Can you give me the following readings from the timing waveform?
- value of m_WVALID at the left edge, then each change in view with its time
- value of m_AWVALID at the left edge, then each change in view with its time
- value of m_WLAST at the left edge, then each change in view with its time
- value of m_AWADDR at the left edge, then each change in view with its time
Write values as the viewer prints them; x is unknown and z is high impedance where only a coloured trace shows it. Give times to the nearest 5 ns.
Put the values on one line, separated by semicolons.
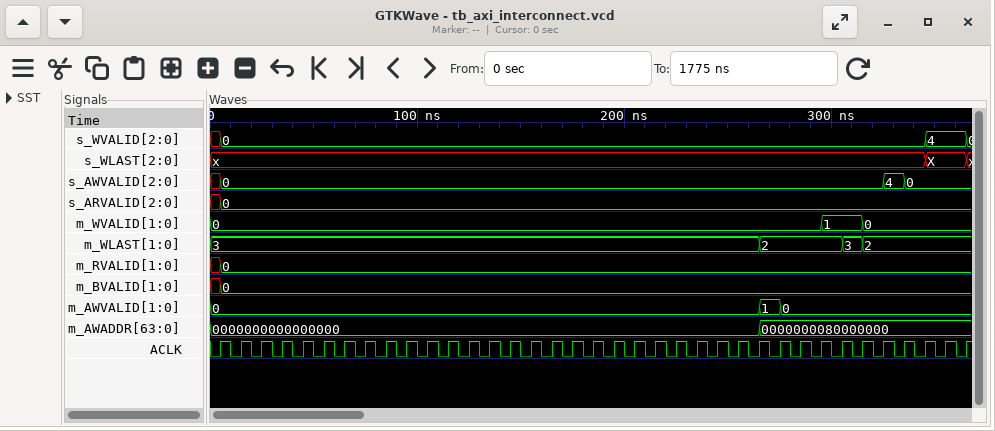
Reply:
0, 1 at 295 ns, 0 at 315 ns; 0, 1 at 265 ns, 0 at 275 ns; 3, 2 at 265 ns, 3 at 305 ns, 2 at 315 ns; 0000000000000000, 0000000080000000 at 265 ns
